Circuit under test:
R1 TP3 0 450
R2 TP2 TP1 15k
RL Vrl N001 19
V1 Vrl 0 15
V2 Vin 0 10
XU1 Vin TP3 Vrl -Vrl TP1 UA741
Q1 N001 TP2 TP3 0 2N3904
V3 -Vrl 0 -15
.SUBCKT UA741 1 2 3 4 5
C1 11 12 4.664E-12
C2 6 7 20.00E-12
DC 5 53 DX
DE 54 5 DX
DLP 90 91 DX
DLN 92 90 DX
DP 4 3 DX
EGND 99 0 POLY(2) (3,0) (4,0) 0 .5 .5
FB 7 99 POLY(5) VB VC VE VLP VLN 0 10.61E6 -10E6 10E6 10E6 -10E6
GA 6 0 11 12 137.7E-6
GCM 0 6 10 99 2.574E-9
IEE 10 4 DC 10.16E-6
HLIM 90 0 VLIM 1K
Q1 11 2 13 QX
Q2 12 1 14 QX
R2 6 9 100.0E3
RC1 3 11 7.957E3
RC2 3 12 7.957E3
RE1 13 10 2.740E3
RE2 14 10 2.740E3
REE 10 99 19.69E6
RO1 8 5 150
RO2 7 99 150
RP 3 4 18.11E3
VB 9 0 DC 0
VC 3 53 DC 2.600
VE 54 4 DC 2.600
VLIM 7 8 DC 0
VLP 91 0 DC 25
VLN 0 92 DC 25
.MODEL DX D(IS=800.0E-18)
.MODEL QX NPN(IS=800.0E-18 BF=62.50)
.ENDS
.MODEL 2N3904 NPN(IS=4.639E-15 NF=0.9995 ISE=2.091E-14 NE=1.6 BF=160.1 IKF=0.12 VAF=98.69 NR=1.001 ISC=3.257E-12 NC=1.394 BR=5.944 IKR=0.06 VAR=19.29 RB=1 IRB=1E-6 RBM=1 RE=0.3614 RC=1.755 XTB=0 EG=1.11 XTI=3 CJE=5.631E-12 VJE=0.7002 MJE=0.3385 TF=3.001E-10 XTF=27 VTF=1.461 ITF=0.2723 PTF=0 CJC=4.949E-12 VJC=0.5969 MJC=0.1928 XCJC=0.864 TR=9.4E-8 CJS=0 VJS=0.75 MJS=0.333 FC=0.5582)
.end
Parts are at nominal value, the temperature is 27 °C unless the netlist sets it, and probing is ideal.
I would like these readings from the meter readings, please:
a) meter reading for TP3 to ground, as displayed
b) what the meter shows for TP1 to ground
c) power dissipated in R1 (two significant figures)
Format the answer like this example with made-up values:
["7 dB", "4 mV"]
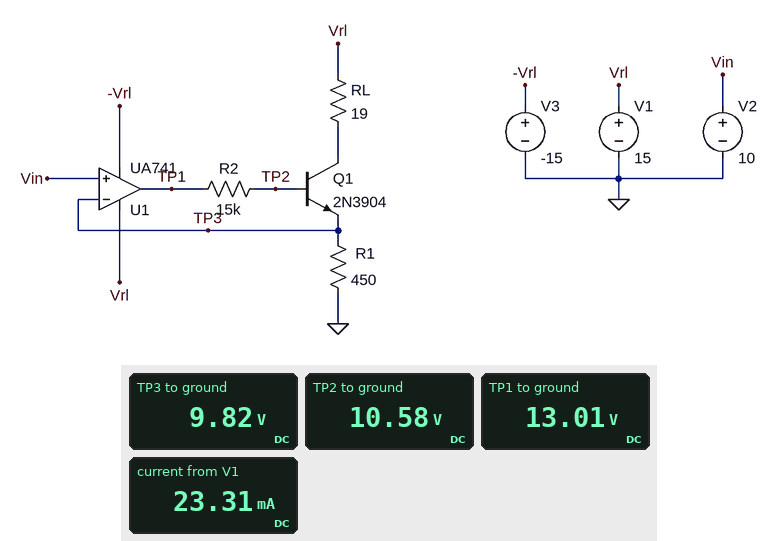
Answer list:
["9.82 V", "13.01 V", "210 mW"]
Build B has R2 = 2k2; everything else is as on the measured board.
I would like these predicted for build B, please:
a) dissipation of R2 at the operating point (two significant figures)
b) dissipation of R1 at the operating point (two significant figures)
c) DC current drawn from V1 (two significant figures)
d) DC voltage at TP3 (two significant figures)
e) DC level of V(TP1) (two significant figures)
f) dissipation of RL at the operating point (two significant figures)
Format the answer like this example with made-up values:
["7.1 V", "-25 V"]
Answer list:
["60 µW", "220 mW", "24 mA", "10 V", "11 V", "9.2 mW"]
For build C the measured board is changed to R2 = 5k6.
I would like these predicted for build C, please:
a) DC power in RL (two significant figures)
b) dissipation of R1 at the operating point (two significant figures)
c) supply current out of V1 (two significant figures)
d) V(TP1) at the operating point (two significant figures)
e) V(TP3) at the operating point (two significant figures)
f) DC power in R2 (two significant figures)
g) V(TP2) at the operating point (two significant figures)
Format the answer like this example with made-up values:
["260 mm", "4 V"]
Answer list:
["9.2 mW", "220 mW", "24 mA", "12 V", "10 V", "150 µW", "11 V"]
